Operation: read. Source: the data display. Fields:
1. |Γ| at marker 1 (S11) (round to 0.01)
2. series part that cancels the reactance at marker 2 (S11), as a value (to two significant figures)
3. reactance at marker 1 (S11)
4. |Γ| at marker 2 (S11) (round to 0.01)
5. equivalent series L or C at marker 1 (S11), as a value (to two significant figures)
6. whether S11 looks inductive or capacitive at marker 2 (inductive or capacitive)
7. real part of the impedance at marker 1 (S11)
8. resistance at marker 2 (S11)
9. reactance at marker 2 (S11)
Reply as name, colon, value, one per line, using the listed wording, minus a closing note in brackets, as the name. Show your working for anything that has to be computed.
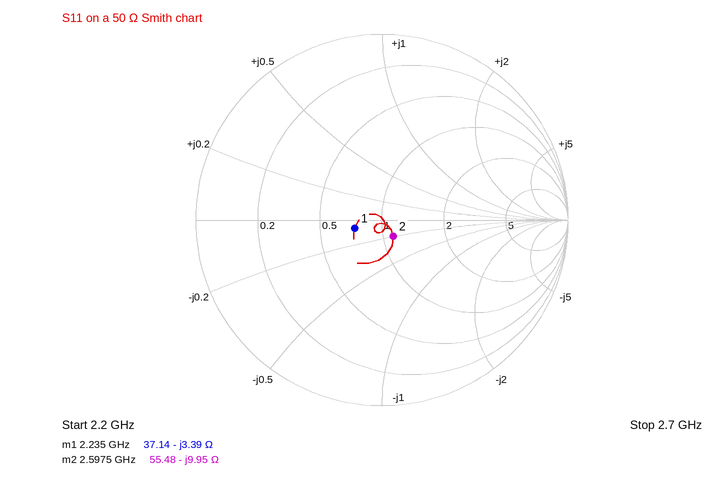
|Γ| at marker 1 (S11): 0.15
series part that cancels the reactance at marker 2 (S11), as a value: L = 9.95 Ω/(2π × 2.5975 GHz) ≈ 610 pH
reactance at marker 1: -3.39 Ω
|Γ| at marker 2 (S11): 0.11
equivalent series L or C at marker 1 (S11), as a value: C = 1/(2π × 2.235 GHz × 3.39 Ω) ≈ 21 pF
whether S11 looks inductive or capacitive at marker 2: capacitive
real part of the impedance at marker 1: 37.14 Ω
resistance at marker 2: 55.48 Ω
reactance at marker 2: -9.95 Ω
